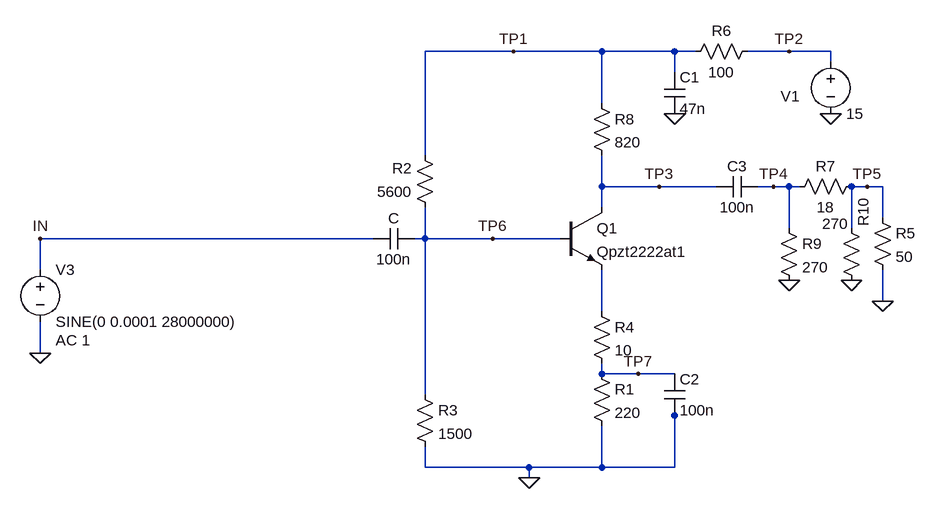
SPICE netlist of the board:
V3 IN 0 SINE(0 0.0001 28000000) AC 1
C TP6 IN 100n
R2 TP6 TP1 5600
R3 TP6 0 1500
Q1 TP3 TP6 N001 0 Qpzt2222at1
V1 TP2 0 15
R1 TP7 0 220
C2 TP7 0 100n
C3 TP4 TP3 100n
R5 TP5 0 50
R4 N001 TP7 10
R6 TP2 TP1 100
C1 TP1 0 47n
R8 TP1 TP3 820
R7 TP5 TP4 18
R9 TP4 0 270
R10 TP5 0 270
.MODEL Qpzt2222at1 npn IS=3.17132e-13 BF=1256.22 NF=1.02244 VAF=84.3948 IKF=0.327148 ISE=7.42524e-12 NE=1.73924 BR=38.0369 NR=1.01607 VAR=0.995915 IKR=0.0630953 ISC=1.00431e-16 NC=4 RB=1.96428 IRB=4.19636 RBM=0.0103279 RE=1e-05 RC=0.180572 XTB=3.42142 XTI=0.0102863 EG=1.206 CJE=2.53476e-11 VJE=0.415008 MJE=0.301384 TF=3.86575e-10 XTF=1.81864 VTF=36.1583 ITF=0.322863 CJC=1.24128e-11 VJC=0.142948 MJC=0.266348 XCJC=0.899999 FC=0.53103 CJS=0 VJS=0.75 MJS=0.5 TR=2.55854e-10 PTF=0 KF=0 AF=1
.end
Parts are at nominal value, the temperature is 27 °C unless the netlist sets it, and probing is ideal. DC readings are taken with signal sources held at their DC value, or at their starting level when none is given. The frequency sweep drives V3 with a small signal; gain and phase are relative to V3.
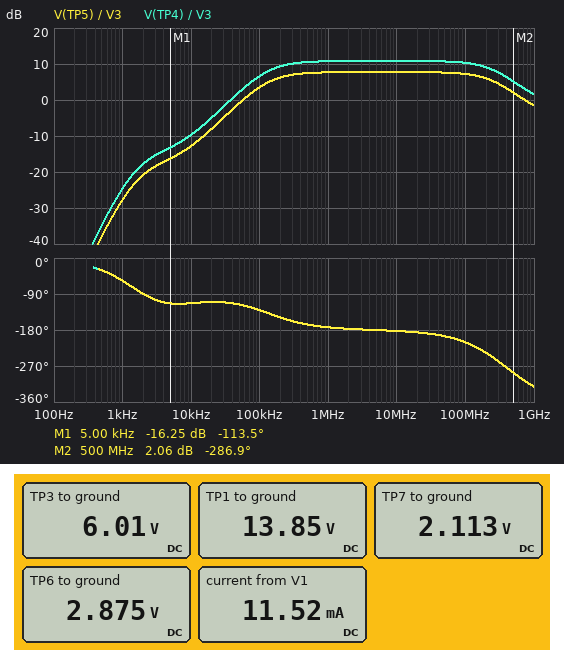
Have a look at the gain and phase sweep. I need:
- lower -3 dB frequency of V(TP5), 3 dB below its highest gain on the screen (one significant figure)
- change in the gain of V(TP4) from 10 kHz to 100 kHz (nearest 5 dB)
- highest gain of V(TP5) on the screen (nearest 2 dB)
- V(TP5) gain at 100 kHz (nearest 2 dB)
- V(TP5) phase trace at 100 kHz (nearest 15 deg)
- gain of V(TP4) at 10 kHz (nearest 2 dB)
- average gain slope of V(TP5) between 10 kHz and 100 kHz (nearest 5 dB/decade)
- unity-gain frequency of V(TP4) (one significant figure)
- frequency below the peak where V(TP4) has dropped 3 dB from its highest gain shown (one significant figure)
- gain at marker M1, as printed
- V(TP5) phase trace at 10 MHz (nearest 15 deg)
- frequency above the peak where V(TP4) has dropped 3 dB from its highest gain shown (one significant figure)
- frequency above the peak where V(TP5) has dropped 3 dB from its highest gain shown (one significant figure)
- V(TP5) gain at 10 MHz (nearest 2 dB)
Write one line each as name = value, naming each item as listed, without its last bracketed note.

lower -3 dB frequency of V(TP5), 3 dB below its highest gain on the screen = 100 kHz
change in the gain of V(TP4) from 10 kHz to 100 kHz = 15 dB
highest gain of V(TP5) on the screen = 8 dB
V(TP5) gain at 100 kHz = 4 dB
V(TP5) phase trace at 100 kHz = -135 deg
gain of V(TP4) at 10 kHz = -10 dB
average gain slope of V(TP5) between 10 kHz and 100 kHz = 15 dB/decade
unity-gain frequency of V(TP4) = 40 kHz
frequency below the peak where V(TP4) has dropped 3 dB from its highest gain shown = 100 kHz
gain at marker M1, as printed = -16.25 dB
V(TP5) phase trace at 10 MHz = -180 deg
frequency above the peak where V(TP4) has dropped 3 dB from its highest gain shown = 300 MHz
frequency above the peak where V(TP5) has dropped 3 dB from its highest gain shown = 300 MHz
V(TP5) gain at 10 MHz = 8 dB
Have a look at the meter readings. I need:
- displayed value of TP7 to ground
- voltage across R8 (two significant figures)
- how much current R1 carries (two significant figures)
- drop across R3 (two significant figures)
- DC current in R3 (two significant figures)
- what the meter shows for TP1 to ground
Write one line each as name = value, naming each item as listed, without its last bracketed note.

displayed value of TP7 to ground = 2.113 V
voltage across R8 = 7.8 V
how much current R1 carries = 9.6 mA
drop across R3 = 2.9 V
DC current in R3 = 1.9 mA
what the meter shows for TP1 to ground = 13.85 V
